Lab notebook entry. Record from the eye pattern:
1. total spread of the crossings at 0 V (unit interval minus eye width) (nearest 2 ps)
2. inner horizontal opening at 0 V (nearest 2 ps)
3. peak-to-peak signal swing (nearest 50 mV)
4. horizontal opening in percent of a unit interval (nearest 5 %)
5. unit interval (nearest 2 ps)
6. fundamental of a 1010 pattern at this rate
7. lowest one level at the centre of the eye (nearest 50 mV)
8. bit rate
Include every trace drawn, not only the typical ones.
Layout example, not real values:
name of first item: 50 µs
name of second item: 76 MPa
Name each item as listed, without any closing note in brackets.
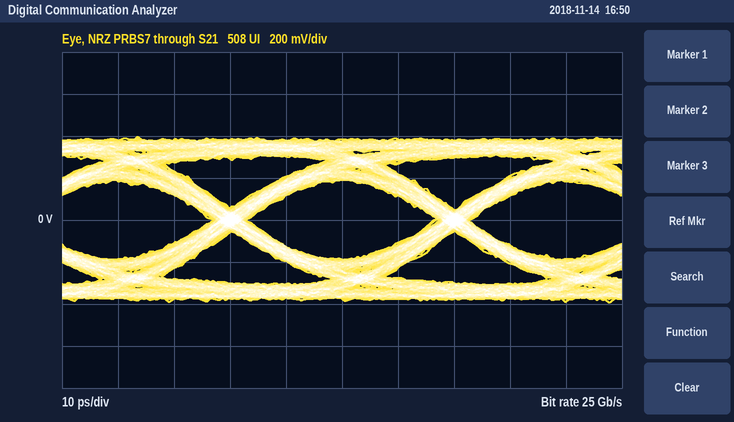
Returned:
total spread of the crossings at 0 V (unit interval minus eye width): 6 ps
inner horizontal opening at 0 V: 34 ps
peak-to-peak signal swing: 800 mV
horizontal opening in percent of a unit interval: 85 %
unit interval: 40 ps
fundamental of a 1010 pattern at this rate: 12.5 GHz
lowest one level at the centre of the eye: 200 mV
bit rate: 25 Gb/s
